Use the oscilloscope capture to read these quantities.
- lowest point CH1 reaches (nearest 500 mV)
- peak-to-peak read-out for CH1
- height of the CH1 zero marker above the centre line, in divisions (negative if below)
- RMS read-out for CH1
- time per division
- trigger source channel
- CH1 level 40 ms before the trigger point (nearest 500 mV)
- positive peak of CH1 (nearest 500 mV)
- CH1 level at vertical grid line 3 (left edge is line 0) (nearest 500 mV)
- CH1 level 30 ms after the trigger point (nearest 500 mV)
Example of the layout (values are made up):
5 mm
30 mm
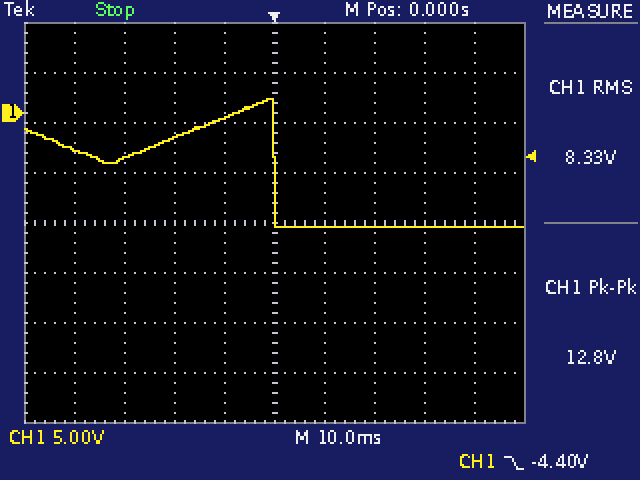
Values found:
-11.5 V
12.8 V
+2.2 div
8.33 V
10 ms
CH1
-3.5 V
1.5 V
-2.5 V
-11.5 V
